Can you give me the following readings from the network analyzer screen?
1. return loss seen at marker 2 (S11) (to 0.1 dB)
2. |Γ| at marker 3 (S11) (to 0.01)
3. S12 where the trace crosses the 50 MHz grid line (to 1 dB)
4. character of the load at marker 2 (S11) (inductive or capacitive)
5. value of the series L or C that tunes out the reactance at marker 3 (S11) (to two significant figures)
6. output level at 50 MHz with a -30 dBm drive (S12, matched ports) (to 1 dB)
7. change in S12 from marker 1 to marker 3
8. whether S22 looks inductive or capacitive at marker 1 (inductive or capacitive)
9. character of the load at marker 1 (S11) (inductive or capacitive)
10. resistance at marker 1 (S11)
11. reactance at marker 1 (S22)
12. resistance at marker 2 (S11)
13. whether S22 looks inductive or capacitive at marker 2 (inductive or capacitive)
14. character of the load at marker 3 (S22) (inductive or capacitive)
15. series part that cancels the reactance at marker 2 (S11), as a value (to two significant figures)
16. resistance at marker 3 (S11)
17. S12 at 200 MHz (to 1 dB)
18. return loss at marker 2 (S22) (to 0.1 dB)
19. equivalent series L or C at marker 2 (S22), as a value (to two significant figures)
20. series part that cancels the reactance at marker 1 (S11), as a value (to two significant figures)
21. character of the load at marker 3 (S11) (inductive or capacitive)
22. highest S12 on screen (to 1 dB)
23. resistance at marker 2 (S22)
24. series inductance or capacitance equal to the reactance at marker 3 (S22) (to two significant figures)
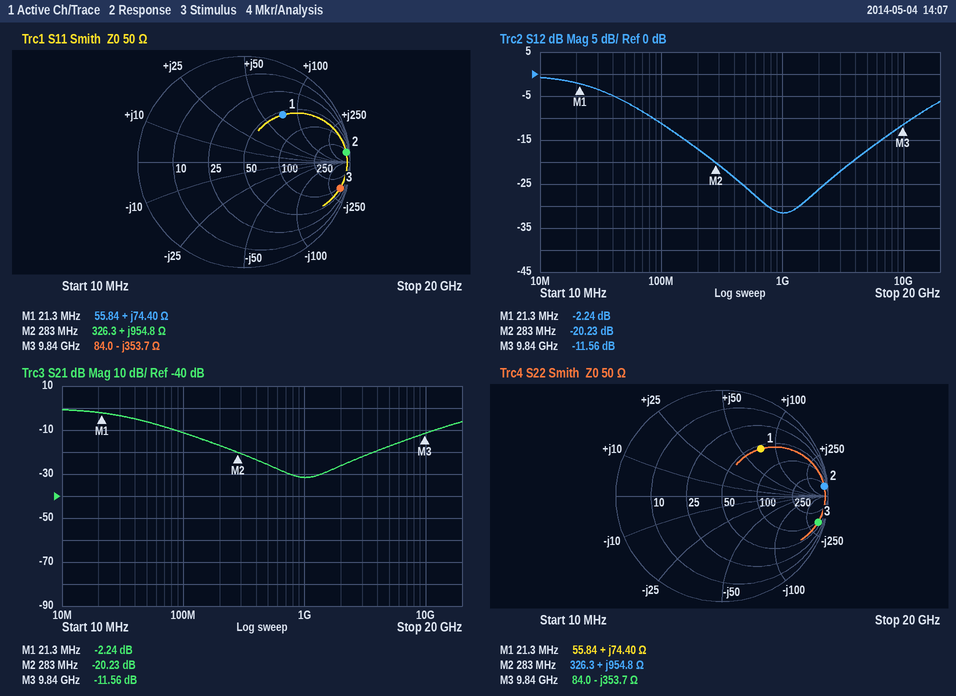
0.3 dB
0.94
-6 dB
inductive
5.7 nH
-36 dBm
-9.32 dB
inductive
inductive
55.84 Ω
+74.40 Ω
326.3 Ω
inductive
capacitive
590 fF
84.0 Ω
-17 dB
0.3 dB
540 nH
100 pF
capacitive
-1 dB
326.3 Ω
46 fF
